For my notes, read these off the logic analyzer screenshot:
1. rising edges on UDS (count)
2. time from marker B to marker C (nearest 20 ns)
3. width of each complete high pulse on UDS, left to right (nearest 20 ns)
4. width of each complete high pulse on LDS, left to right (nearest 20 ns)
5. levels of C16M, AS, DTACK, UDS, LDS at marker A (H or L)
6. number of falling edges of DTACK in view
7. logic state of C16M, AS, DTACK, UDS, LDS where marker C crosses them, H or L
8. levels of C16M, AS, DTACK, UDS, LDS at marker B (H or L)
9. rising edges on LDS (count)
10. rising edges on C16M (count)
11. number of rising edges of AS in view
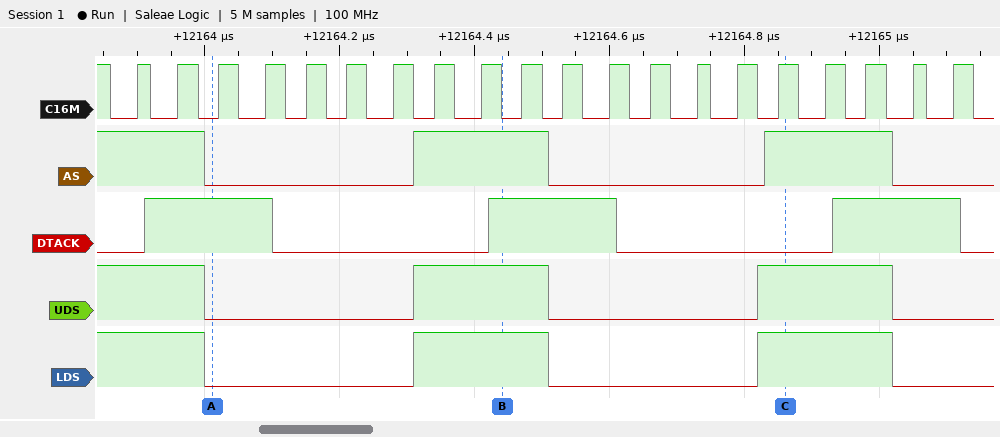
2
420 ns
200 ns, 200 ns
200 ns, 200 ns
C16M=L, AS=L, DTACK=H, UDS=L, LDS=L
3
C16M=H, AS=H, DTACK=L, UDS=H, LDS=H
C16M=L, AS=H, DTACK=H, UDS=H, LDS=H
2
20
2
